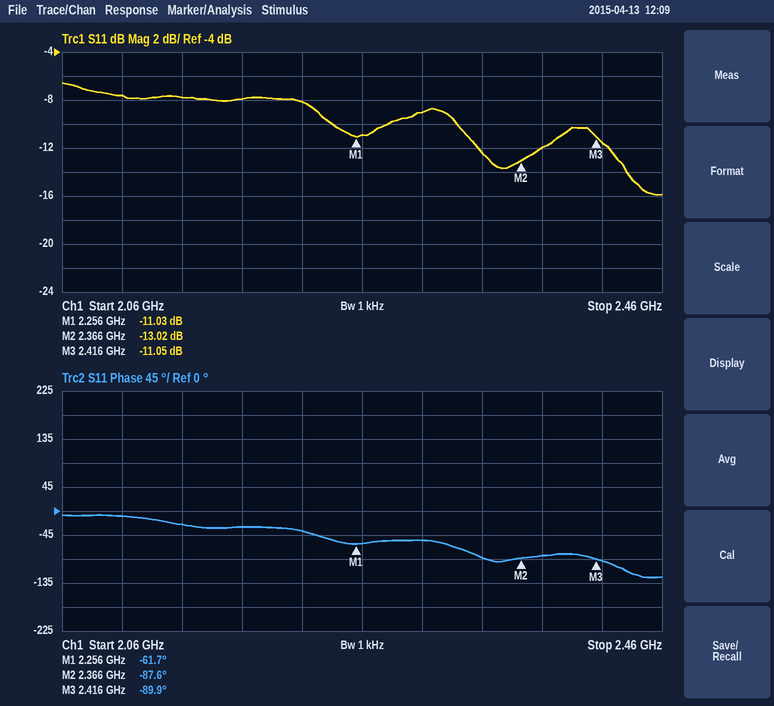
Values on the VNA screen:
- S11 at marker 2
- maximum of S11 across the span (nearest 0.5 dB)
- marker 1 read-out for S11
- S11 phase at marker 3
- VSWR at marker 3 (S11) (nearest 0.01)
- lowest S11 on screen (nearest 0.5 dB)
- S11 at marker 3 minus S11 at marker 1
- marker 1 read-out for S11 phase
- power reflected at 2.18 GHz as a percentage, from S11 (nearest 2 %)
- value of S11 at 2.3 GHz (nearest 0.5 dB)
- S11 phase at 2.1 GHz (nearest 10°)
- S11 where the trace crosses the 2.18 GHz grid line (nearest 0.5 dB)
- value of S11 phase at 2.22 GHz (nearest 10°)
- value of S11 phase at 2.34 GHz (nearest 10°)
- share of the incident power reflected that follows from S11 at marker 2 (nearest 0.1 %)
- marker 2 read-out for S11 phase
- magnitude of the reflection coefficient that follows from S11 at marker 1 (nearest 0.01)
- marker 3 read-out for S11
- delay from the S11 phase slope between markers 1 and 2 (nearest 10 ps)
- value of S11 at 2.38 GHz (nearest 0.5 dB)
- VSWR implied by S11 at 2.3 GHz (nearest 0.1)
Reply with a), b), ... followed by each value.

a) -13.02 dB
b) -6.5 dB
c) -11.03 dB
d) -89.9°
e) 1.78
f) -16.0 dB
g) -0.02 dB
h) -61.7°
i) 16 %
j) -9.0 dB
k) -10°
l) -8.0 dB
m) -40°
n) -90°
o) 5.0 %
p) -87.6°
q) 0.28
r) -11.05 dB
s) 650 ps
t) -12.0 dB
u) 2.1
